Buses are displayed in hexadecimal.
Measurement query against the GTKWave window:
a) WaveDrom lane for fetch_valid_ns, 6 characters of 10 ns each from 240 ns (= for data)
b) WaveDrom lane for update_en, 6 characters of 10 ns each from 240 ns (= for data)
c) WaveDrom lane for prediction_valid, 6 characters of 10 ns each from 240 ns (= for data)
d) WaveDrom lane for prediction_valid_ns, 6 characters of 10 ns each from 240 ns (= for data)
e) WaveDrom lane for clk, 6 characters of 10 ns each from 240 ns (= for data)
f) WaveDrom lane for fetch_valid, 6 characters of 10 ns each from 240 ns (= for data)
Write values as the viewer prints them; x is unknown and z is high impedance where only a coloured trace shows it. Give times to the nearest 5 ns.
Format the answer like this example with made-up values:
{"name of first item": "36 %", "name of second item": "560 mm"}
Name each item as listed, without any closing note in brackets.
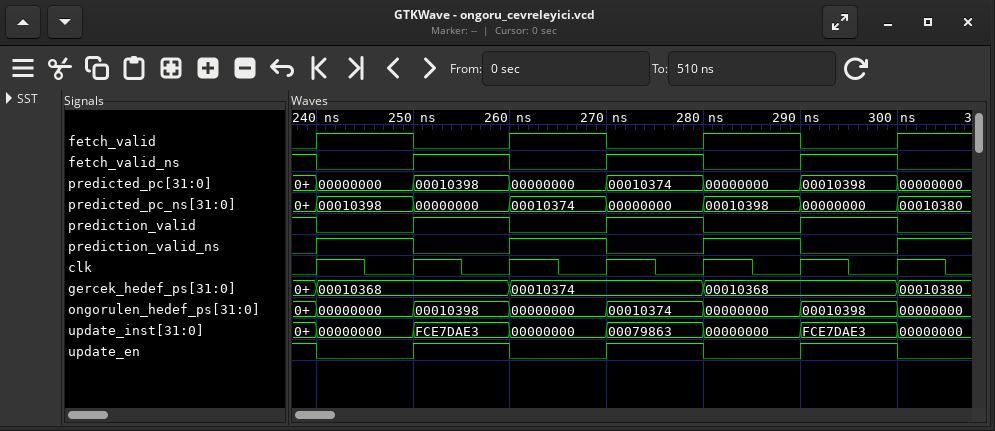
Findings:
{"WaveDrom lane for fetch_valid_ns, 6 characters of 10 ns each from 240 ns": "{name: 'fetch_valid_ns', wave: '010101'}", "WaveDrom lane for update_en, 6 characters of 10 ns each from 240 ns": "{name: 'update_en', wave: '010101'}", "WaveDrom lane for prediction_valid, 6 characters of 10 ns each from 240 ns": "{name: 'prediction_valid', wave: '010101'}", "WaveDrom lane for prediction_valid_ns, 6 characters of 10 ns each from 240 ns": "{name: 'prediction_valid_ns', wave: '101010'}", "WaveDrom lane for clk, 6 characters of 10 ns each from 240 ns": "{name: 'clk', wave: 'p.....'}", "WaveDrom lane for fetch_valid, 6 characters of 10 ns each from 240 ns": "{name: 'fetch_valid', wave: '101010'}"}
